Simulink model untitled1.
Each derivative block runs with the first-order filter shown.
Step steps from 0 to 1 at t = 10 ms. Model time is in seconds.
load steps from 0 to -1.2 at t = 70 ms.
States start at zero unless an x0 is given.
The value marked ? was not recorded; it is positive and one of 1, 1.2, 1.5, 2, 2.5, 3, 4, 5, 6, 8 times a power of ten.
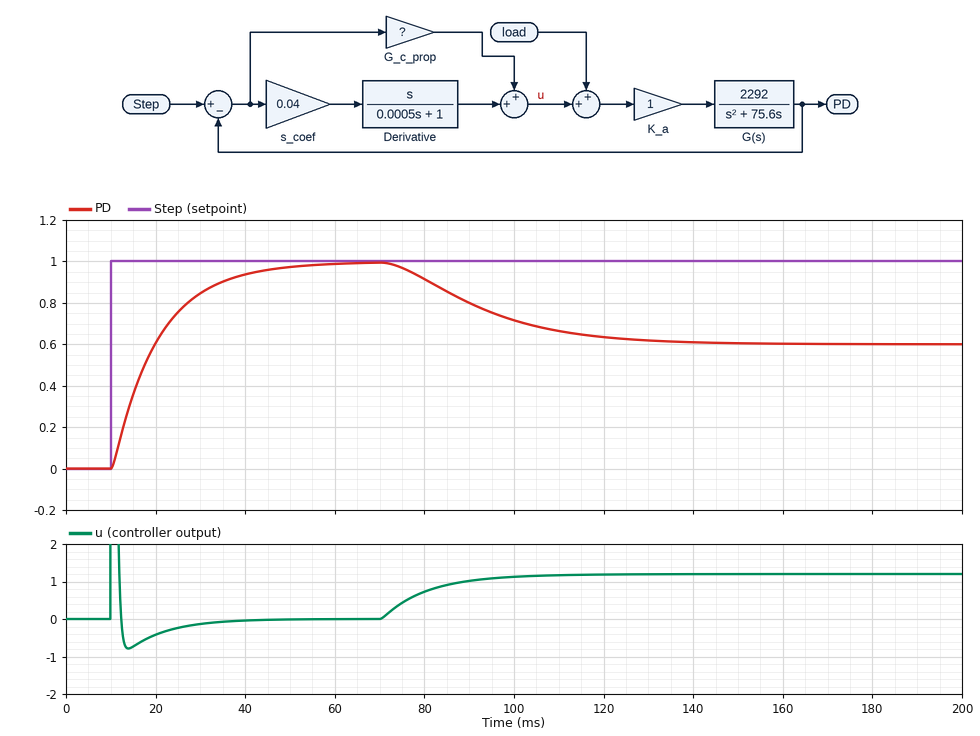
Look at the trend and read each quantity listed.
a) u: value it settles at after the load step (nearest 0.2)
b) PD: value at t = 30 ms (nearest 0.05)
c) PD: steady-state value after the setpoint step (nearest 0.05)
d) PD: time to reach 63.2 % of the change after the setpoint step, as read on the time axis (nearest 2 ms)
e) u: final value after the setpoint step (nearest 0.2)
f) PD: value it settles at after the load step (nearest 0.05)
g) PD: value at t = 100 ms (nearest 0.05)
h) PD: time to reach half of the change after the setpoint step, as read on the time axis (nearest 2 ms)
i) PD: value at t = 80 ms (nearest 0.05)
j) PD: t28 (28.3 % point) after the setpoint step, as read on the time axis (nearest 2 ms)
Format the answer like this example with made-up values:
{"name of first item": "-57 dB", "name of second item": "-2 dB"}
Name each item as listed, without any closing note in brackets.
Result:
{"u: value it settles at after the load step": "1.2", "PD: value at t = 30 ms": "0.85", "PD: steady-state value after the setpoint step": "1.00", "PD: time to reach 63.2 % of the change after the setpoint step, as read on the time axis": "20 ms", "u: final value after the setpoint step": "0.0", "PD: value it settles at after the load step": "0.60", "PD: value at t = 100 ms": "0.70", "PD: time to reach half of the change after the setpoint step, as read on the time axis": "18 ms", "PD: value at t = 80 ms": "0.90", "PD: t28 (28.3 % point) after the setpoint step, as read on the time axis": "14 ms"}
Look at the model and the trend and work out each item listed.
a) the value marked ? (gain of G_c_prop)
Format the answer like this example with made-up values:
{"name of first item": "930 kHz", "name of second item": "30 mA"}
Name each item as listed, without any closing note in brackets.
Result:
{"the value marked ?": "3"}
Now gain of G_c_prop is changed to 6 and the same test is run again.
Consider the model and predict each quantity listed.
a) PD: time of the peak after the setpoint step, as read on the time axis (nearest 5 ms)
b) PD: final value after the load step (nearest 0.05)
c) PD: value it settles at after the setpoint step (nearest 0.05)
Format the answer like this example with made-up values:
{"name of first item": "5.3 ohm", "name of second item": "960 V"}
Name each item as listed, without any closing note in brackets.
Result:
{"PD: time of the peak after the setpoint step, as read on the time axis": "35 ms", "PD: final value after the load step": "0.80", "PD: value it settles at after the setpoint step": "1.00"}
